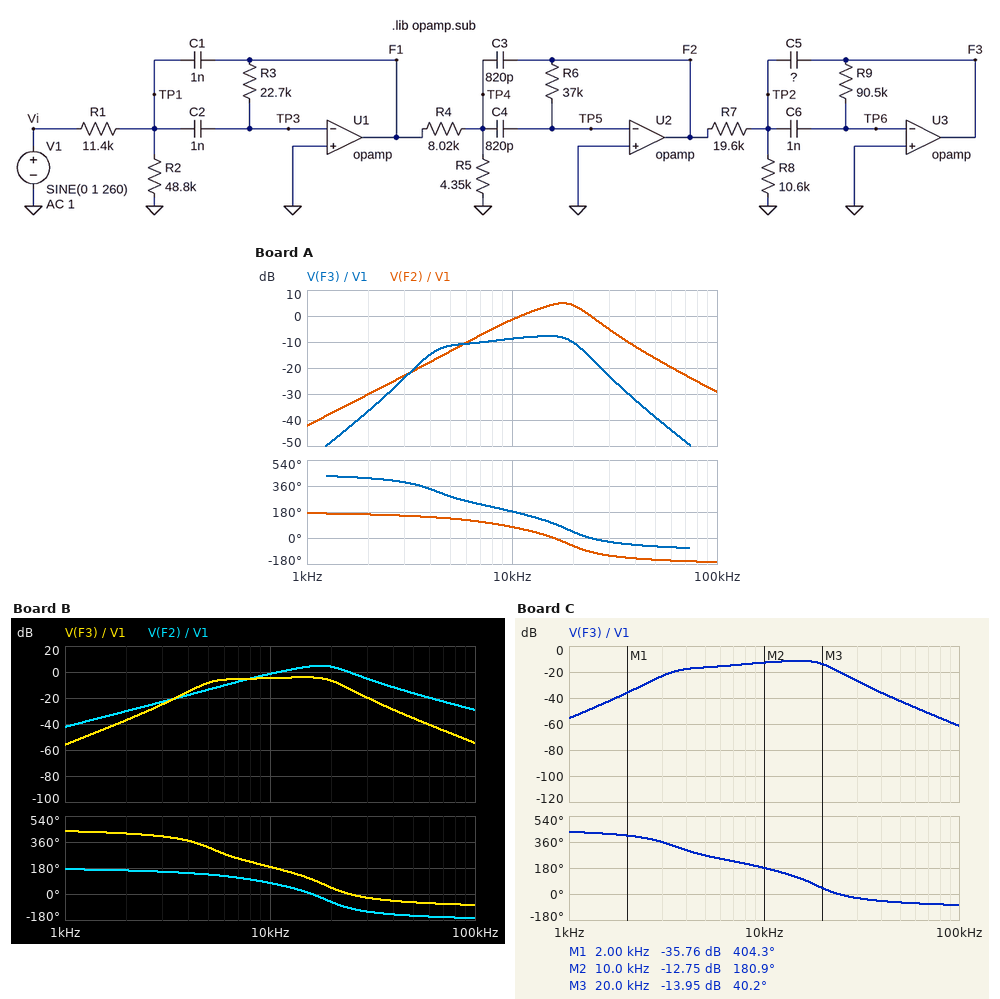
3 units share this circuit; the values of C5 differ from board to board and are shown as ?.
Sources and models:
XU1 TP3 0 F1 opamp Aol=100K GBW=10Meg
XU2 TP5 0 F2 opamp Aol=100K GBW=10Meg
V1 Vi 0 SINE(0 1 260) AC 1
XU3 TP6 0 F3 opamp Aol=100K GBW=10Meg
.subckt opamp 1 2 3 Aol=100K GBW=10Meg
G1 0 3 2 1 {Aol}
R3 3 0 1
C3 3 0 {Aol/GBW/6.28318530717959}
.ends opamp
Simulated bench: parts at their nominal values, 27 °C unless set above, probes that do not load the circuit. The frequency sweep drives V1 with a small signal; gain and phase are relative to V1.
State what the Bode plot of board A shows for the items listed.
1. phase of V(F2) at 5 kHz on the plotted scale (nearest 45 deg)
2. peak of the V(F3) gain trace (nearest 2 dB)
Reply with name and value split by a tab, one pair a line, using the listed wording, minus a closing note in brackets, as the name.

phase of V(F2) at 5 kHz on the plotted scale	135 deg
peak of the V(F3) gain trace	-8 dB
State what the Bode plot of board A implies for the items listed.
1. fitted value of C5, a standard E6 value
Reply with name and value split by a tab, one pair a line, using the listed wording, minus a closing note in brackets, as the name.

fitted value of C5, a standard E6 value	2.2 nF
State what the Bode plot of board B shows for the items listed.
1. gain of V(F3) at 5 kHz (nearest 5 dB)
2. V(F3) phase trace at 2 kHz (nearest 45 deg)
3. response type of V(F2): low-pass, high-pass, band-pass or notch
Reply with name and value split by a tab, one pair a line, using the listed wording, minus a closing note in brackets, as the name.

gain of V(F3) at 5 kHz	-10 dB
V(F3) phase trace at 2 kHz	405 deg
response type of V(F2): low-pass, high-pass, band-pass or notch	band-pass
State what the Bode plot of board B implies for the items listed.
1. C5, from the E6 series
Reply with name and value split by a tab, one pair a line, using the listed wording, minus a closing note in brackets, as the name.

C5, from the E6 series	1.5 nF
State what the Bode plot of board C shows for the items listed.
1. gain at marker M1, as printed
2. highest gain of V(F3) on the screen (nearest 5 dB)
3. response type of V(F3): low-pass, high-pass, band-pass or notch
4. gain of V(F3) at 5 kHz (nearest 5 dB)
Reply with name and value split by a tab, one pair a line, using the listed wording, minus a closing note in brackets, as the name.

gain at marker M1, as printed	-35.76 dB
highest gain of V(F3) on the screen	-10 dB
response type of V(F3): low-pass, high-pass, band-pass or notch	band-pass
gain of V(F3) at 5 kHz	-15 dB
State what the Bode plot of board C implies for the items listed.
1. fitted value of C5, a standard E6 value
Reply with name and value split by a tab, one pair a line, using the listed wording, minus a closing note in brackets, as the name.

fitted value of C5, a standard E6 value	3.3 nF
